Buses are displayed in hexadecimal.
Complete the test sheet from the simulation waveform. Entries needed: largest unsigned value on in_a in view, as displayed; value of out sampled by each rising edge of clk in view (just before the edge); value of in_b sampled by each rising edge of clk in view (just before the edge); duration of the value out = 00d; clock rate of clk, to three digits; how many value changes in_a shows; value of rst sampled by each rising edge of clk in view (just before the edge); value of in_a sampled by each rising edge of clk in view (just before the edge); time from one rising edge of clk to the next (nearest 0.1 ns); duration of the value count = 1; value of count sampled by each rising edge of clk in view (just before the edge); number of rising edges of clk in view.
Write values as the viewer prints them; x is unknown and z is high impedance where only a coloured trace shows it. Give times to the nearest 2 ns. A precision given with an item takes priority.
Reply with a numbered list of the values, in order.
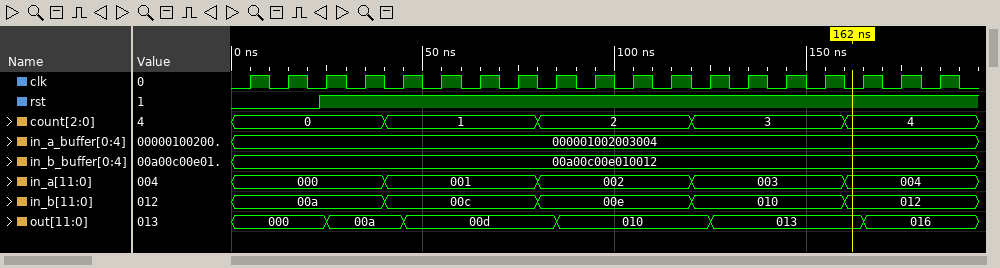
1. 004
2. 000, 000, 000, 00a, 00a, 00d, 00d, 00d, 00d, 010, 010, 010, 010, 013, 013, 013, 013, 016, 016
3. 00a, 00a, 00a, 00a, 00c, 00c, 00c, 00c, 00e, 00e, 00e, 00e, 010, 010, 010, 010, 012, 012, 012
4. 40 ns
5. 100 MHz
6. 4
7. 0 0 1 1 1 1 1 1 1 1 1 1 1 1 1 1 1 1 1
8. 000, 000, 000, 000, 001, 001, 001, 001, 002, 002, 002, 002, 003, 003, 003, 003, 004, 004, 004
9. 10 ns
10. 40 ns
11. 0, 0, 0, 0, 1, 1, 1, 1, 2, 2, 2, 2, 3, 3, 3, 3, 4, 4, 4
12. 19
